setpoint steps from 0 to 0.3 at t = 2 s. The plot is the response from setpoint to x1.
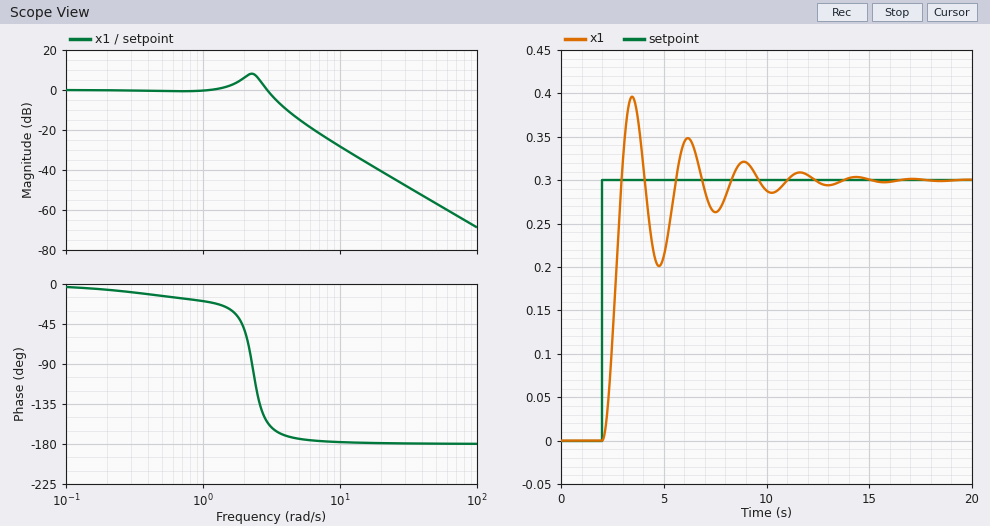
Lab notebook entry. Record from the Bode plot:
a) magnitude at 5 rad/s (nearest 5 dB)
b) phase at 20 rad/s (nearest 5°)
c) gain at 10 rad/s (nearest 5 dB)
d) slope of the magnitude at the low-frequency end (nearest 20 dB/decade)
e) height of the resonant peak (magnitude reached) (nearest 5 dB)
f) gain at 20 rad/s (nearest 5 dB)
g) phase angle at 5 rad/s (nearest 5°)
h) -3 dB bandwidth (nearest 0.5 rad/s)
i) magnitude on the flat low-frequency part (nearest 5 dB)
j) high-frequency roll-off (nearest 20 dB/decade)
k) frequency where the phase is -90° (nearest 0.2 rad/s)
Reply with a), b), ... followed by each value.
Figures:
a) -15 dB
b) -180°
c) -30 dB
d) 0 dB/decade
e) 10 dB
f) -40 dB
g) -175°
h) 3.0 rad/s
i) 0 dB
j) -40 dB/decade
k) 2.2 rad/s
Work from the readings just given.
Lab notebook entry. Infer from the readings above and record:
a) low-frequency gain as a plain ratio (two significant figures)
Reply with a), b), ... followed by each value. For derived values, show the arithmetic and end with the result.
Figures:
a) 10^(0 / 20) = 1.0
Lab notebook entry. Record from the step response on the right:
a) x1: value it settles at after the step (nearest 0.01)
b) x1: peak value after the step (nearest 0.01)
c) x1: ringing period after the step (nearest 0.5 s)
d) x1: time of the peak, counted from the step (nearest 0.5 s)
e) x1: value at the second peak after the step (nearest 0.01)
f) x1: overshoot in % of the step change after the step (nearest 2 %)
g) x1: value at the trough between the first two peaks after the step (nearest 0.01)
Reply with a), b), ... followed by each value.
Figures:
a) 0.30
b) 0.40
c) 2.5 s
d) 1.5 s
e) 0.35
f) 32 %
g) 0.20
